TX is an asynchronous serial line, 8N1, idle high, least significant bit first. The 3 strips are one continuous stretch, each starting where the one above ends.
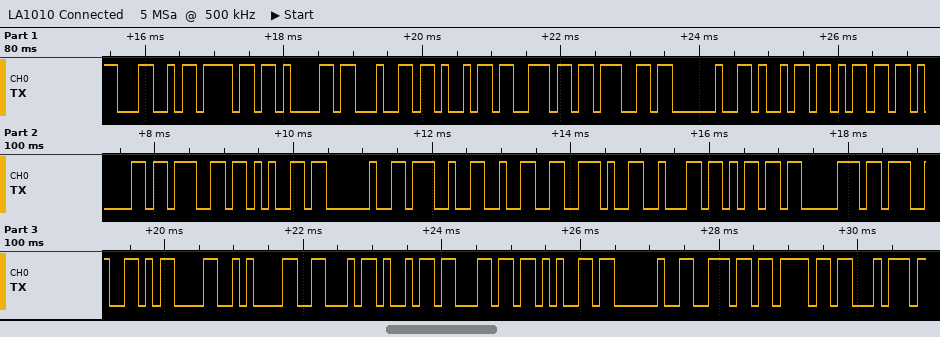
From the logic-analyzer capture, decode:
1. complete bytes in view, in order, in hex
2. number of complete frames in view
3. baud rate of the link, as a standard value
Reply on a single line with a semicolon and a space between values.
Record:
0x4C 0x6F 0x61 0x64 0x69 0x6E 0x67 0x20 0x69 0x6D 0x61 0x67 0x65 0x20 0x27 0x32 0x2E 0x62 0x6D 0x70 0x27 0x0D 0x0A 0x46 0x69 0x6C 0x65 0x20 0x6E 0x6F 0x74; 31; 9600 baud
